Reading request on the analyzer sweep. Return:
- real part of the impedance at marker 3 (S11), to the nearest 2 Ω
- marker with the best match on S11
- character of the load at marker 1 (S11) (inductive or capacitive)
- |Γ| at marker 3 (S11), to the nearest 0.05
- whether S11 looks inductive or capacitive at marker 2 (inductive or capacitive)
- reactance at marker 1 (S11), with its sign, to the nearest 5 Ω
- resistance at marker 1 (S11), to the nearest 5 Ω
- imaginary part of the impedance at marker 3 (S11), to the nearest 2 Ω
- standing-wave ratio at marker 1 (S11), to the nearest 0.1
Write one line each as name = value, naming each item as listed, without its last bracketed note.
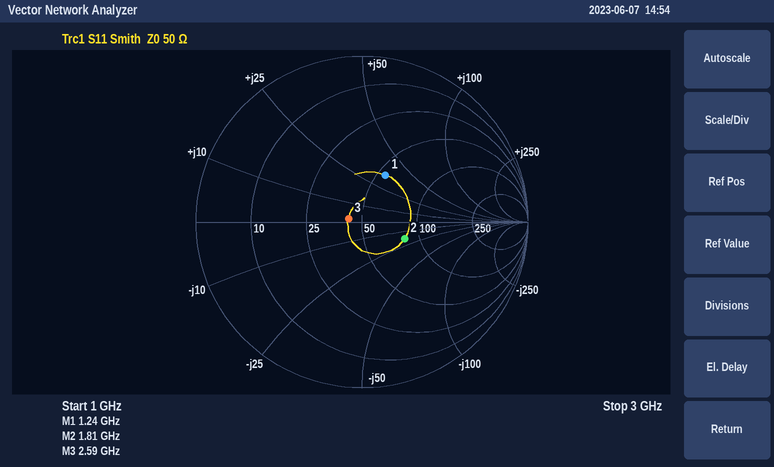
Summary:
real part of the impedance at marker 3 (S11), to the nearest 2 Ω = 42 Ω
marker with the best match on S11 = marker 3
character of the load at marker 1 (S11) = inductive
|Γ| at marker 3 (S11), to the nearest 0.05 = 0.10
whether S11 looks inductive or capacitive at marker 2 = capacitive
reactance at marker 1 (S11), with its sign, to the nearest 5 Ω = +35 Ω
resistance at marker 1 (S11), to the nearest 5 Ω = 55 Ω
imaginary part of the impedance at marker 3 (S11), to the nearest 2 Ω = +2 Ω
standing-wave ratio at marker 1 (S11), to the nearest 0.1 = 1.9
